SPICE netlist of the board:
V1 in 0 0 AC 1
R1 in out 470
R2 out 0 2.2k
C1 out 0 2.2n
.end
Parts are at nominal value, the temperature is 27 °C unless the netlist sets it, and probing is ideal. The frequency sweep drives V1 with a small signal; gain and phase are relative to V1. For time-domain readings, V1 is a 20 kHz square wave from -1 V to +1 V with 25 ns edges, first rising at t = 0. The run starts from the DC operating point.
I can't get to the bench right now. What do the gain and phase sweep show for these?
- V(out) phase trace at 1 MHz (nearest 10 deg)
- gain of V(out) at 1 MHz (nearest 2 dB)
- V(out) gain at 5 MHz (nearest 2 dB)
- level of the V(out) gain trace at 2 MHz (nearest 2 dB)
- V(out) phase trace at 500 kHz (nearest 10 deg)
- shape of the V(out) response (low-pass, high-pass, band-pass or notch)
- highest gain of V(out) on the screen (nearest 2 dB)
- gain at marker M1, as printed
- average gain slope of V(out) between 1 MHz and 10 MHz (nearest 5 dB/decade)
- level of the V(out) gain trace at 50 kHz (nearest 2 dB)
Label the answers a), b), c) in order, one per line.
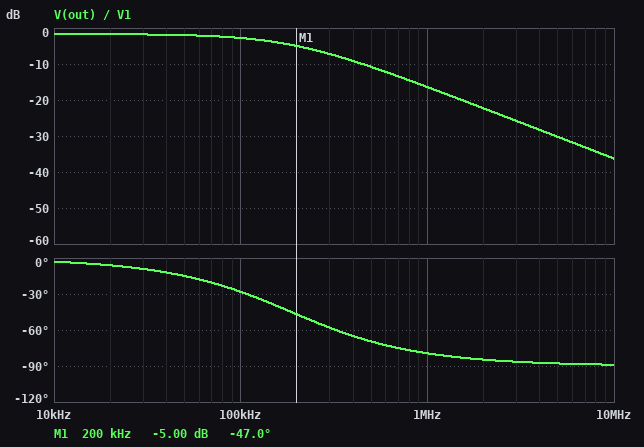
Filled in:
a) -80 deg
b) -16 dB
c) -30 dB
d) -22 dB
e) -70 deg
f) low-pass
g) -2 dB
h) -5.00 dB
i) -20 dB/decade
j) -2 dB
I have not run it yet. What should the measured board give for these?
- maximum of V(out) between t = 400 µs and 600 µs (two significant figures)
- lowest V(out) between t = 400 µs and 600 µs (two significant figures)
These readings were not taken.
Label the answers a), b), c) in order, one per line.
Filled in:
a) 820 mV
b) -820 mV
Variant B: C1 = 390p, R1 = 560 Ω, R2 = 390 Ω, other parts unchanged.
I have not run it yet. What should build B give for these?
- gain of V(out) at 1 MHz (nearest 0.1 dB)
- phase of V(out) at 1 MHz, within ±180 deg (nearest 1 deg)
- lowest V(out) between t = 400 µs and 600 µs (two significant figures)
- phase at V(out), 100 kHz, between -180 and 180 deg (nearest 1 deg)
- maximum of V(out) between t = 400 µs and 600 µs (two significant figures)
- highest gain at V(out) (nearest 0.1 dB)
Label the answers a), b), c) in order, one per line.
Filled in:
a) -8.9 dB
b) -29 deg
c) -410 mV
d) -3 deg
e) 410 mV
f) -7.7 dB
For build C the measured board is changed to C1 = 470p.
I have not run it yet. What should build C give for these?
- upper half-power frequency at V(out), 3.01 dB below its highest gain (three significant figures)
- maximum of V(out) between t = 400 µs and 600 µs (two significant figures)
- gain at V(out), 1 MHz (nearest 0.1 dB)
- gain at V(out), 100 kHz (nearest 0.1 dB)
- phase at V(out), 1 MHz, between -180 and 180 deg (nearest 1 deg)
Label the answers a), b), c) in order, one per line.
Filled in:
a) 874 kHz
b) 820 mV
c) -5.3 dB
d) -1.7 dB
e) -49 deg
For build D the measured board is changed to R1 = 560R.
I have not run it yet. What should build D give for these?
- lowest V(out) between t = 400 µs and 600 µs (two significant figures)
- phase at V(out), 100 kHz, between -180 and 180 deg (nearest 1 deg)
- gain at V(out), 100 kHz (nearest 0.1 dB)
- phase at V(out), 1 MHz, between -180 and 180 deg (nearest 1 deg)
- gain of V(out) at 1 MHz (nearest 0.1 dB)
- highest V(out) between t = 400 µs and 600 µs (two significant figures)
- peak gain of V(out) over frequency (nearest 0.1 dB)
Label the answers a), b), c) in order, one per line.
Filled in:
a) -800 mV
b) -32 deg
c) -3.4 dB
d) -81 deg
e) -17.9 dB
f) 800 mV
g) -2.0 dB
